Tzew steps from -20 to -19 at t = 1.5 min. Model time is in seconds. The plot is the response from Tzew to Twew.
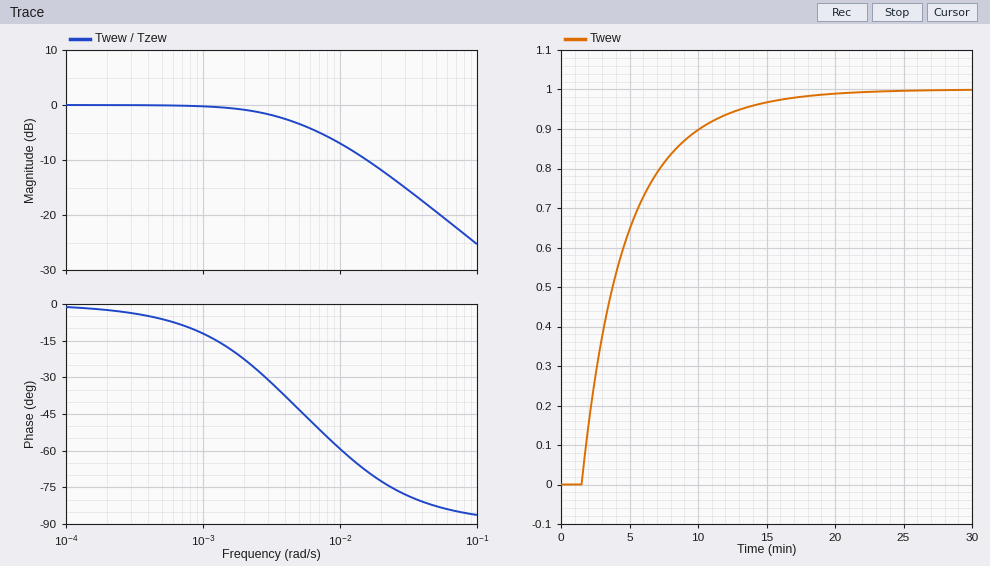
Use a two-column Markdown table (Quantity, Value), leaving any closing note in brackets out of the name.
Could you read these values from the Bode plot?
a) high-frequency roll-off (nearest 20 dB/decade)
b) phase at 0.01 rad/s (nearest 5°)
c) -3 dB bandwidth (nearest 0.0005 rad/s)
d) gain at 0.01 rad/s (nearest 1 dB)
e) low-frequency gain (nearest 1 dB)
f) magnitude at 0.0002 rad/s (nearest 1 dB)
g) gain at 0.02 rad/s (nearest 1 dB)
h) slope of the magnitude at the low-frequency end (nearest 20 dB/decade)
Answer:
| Quantity | Value |
|---|---|
| high-frequency roll-off | -20 dB/decade |
| phase at 0.01 rad/s | -60° |
| -3 dB bandwidth | 0.0045 rad/s |
| gain at 0.01 rad/s | -7 dB |
| low-frequency gain | 0 dB |
| magnitude at 0.0002 rad/s | 0 dB |
| gain at 0.02 rad/s | -12 dB |
| slope of the magnitude at the low-frequency end | 0 dB/decade |
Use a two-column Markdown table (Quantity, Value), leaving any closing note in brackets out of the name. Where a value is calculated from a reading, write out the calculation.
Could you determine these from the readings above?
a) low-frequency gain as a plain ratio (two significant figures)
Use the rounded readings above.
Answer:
| Quantity | Value |
|---|---|
| low-frequency gain as a plain ratio | 10^(0 / 20) = 1.0 |
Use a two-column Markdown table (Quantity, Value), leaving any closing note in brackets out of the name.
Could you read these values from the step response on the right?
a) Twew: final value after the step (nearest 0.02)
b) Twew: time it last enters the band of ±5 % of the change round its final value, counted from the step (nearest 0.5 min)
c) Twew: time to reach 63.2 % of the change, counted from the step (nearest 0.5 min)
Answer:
| Quantity | Value |
|---|---|
| Twew: final value after the step | 1.00 |
| Twew: time it last enters the band of ±5 % of the change round its final value, counted from the step | 11.5 min |
| Twew: time to reach 63.2 % of the change, counted from the step | 3.5 min |
